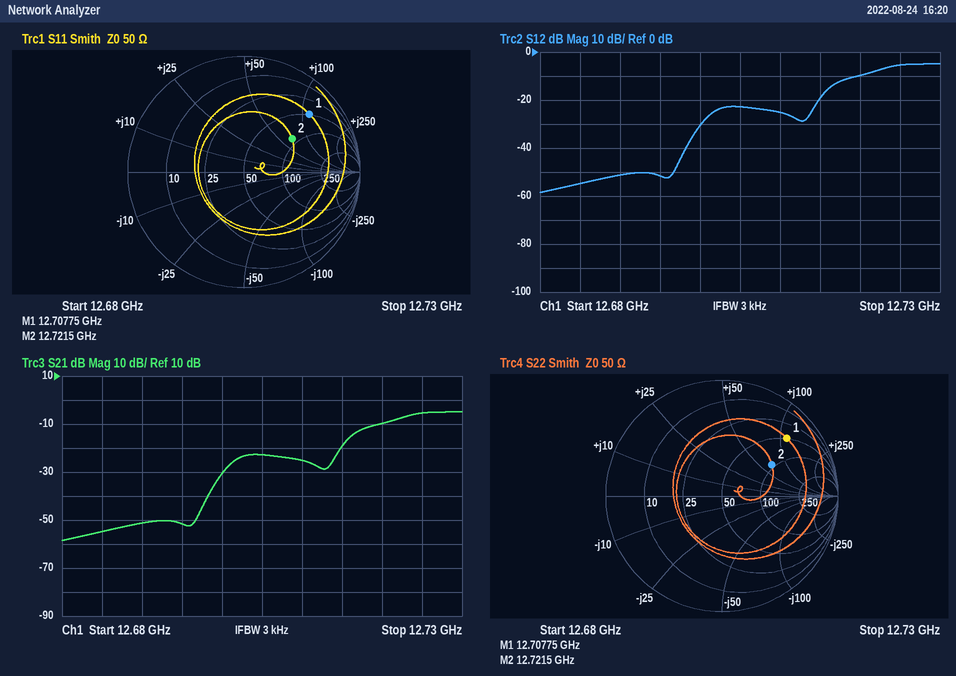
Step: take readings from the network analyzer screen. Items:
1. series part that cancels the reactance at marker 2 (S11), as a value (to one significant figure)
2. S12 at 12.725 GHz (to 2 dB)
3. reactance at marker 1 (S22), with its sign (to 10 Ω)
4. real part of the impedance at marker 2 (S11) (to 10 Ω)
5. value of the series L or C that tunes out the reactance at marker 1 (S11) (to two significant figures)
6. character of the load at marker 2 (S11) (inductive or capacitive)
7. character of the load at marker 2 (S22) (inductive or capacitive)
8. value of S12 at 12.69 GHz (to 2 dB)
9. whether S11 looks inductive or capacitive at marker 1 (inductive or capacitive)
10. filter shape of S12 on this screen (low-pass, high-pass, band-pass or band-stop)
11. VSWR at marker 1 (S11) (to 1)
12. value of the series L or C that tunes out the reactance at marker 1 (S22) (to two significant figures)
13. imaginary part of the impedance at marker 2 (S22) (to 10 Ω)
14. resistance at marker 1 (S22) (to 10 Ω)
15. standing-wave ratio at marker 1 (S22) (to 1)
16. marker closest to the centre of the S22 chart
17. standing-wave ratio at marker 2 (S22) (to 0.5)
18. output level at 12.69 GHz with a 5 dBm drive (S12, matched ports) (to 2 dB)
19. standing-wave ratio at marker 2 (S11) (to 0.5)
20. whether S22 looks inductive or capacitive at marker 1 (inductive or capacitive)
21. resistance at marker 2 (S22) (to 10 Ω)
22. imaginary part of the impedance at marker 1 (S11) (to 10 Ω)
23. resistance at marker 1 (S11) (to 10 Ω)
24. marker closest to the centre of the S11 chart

200 fF
-6 dB
+110 Ω
90 Ω
110 fF
inductive
inductive
-52 dB
inductive
high-pass
7
110 fF
+70 Ω
50 Ω
7
marker 2
3.0
-46 dBm
3.0
inductive
90 Ω
+110 Ω
50 Ω
marker 2
